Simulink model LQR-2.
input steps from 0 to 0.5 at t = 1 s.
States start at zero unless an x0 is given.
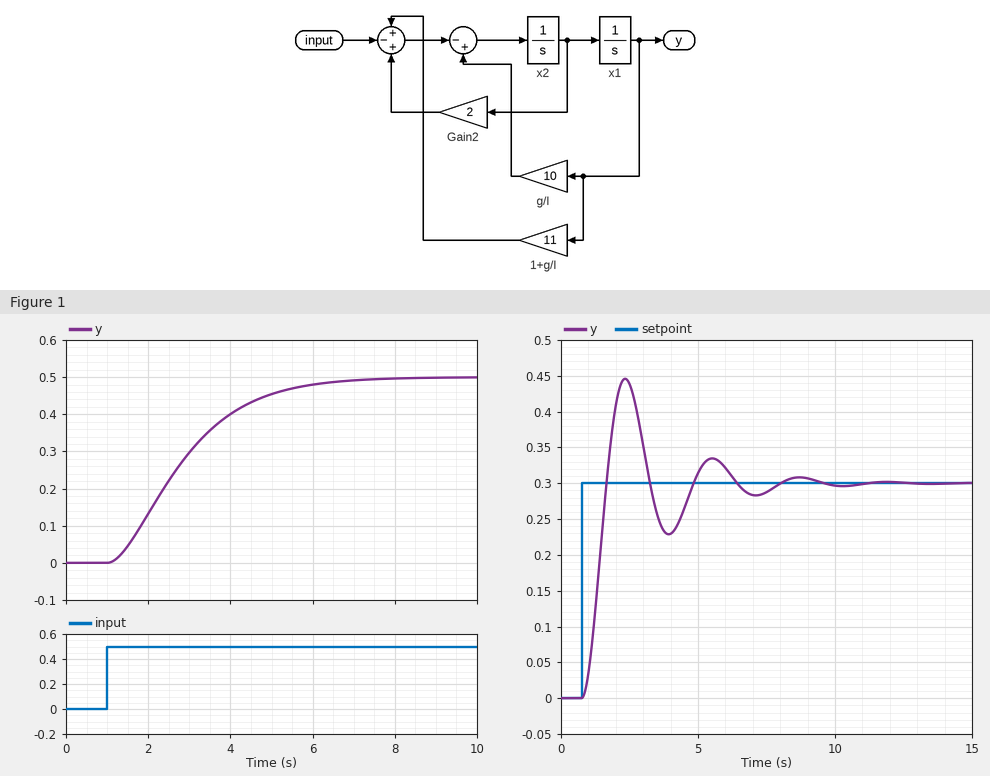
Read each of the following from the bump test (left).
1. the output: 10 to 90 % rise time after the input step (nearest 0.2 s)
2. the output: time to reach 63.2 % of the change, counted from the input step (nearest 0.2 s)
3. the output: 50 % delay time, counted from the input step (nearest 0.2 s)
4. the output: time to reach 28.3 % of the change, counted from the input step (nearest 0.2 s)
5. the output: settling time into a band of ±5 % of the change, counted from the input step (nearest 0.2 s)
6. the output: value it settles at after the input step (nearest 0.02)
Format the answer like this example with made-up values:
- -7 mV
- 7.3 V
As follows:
- 3.4 s
- 2.2 s
- 1.6 s
- 1.0 s
- 4.8 s
- 0.50
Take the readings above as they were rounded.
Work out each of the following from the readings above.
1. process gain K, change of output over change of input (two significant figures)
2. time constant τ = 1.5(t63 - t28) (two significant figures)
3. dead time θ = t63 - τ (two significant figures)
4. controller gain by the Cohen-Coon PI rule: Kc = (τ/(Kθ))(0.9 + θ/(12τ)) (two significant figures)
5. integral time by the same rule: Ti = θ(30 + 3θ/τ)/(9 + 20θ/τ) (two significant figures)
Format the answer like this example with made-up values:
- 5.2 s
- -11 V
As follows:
- 1.0
- 1.8 s
- 0.40 s
- 4.1
- 0.91 s
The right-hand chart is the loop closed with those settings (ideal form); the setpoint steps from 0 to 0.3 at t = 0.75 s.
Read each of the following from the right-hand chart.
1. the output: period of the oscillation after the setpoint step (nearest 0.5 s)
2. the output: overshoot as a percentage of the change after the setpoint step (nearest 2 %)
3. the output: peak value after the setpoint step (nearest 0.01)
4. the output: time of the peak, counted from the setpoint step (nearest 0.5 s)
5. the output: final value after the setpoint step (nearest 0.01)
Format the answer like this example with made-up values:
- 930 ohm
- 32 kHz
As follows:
- 3.0 s
- 48 %
- 0.45
- 1.5 s
- 0.30
